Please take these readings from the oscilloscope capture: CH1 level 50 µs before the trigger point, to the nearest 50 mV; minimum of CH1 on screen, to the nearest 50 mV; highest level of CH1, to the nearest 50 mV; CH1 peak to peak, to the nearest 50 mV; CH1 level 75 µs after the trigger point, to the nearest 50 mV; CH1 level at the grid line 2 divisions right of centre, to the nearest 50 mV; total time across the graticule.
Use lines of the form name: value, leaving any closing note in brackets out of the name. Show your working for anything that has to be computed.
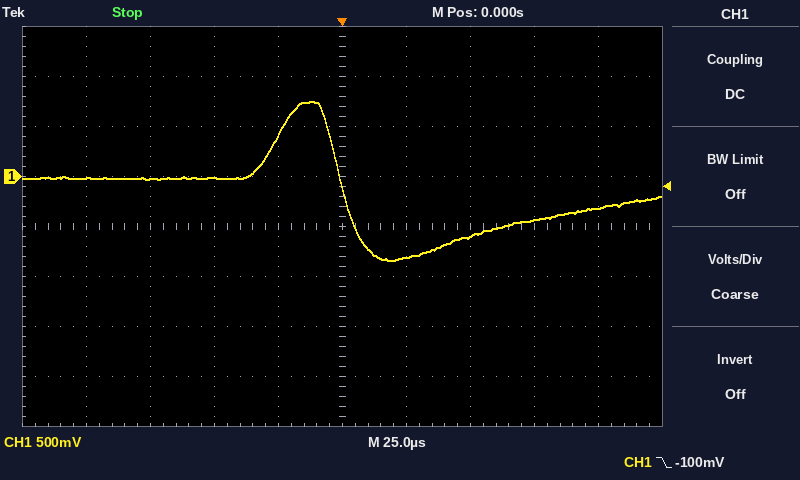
CH1 level 50 µs before the trigger point, to the nearest 50 mV: 0 mV
minimum of CH1 on screen, to the nearest 50 mV: -850 mV
highest level of CH1, to the nearest 50 mV: 750 mV
CH1 peak to peak, to the nearest 50 mV: 750 mV − (-850 mV) = 1.60 V
CH1 level 75 µs after the trigger point, to the nearest 50 mV: -450 mV
CH1 level at the grid line 2 divisions right of centre, to the nearest 50 mV: -600 mV
total time across the graticule: 250 µs
